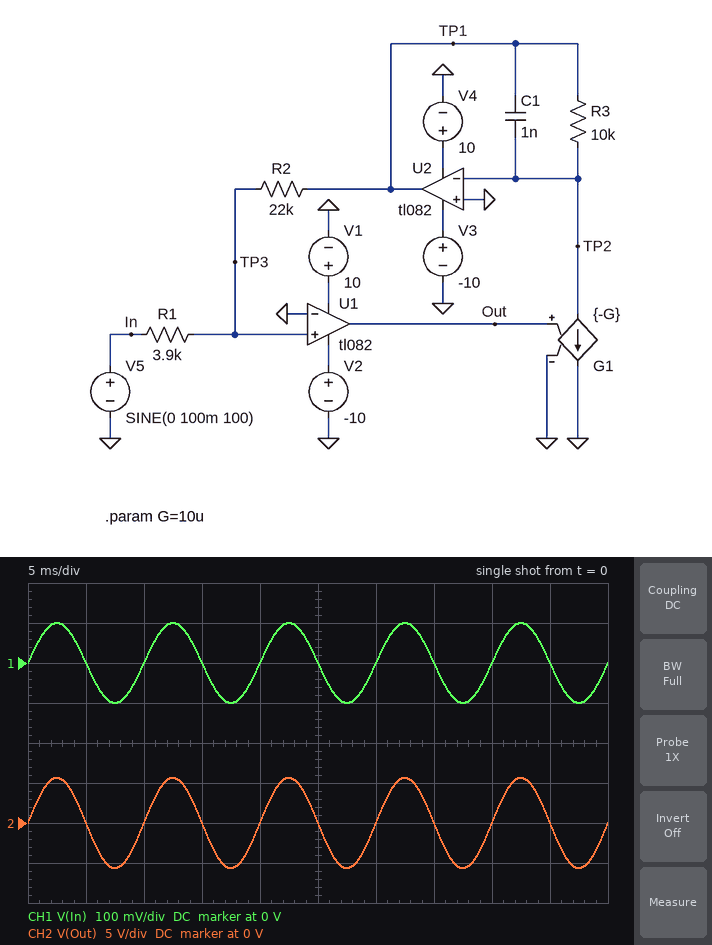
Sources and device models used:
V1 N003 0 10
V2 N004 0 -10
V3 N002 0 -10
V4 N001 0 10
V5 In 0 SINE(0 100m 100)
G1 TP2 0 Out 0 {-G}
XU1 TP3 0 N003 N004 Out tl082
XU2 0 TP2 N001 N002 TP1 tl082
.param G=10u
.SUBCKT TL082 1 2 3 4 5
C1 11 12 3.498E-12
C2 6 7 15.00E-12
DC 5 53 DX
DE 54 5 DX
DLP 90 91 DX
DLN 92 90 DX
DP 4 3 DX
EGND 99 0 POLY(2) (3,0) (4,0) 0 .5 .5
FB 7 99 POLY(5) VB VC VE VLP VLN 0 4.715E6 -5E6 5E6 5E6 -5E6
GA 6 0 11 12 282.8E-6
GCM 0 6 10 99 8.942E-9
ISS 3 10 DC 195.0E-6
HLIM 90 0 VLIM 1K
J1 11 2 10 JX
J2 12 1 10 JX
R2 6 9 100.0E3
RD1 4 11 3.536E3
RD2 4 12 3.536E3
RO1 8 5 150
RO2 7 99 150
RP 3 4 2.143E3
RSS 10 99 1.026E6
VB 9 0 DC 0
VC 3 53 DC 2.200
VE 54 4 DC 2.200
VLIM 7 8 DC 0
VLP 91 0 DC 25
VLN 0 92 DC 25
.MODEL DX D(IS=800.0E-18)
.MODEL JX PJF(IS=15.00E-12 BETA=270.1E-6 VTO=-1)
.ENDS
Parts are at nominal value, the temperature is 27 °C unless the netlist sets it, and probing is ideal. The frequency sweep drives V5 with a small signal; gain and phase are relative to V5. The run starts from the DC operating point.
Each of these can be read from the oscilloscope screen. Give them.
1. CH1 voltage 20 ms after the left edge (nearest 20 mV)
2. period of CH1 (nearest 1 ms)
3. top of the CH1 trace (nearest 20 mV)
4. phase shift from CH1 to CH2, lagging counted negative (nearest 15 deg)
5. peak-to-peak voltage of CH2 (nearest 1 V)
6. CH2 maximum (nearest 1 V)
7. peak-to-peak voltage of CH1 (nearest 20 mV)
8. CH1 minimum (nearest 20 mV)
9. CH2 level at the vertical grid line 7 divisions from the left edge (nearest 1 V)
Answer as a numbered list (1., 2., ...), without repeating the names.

1. 0 V
2. 10 ms
3. 100 mV
4. 0 deg
5. 11 V
6. 6 V
7. 200 mV
8. -100 mV
9. 0 V
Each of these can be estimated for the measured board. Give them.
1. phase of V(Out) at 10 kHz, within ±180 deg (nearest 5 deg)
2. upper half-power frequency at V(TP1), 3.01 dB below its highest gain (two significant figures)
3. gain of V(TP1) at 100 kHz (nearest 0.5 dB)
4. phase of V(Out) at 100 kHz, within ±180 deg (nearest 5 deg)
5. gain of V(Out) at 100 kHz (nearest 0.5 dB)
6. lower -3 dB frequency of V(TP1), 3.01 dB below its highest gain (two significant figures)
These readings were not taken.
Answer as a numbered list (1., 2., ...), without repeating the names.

1. 20 deg
2. 34 kHz
3. -6.0 dB
4. -90 deg
5. 30.0 dB
6. 17 kHz
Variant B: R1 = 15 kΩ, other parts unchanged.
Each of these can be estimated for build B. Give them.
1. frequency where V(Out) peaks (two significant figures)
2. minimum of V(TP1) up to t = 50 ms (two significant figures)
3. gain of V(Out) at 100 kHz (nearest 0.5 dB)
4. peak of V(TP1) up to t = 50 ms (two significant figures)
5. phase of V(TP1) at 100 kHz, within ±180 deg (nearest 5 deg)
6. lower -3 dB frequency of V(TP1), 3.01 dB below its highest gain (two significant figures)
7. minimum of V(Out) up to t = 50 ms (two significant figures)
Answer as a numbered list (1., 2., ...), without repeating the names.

1. 47 kHz
2. -150 mV
3. 28.5 dB
4. 150 mV
5. 10 deg
6. 38 kHz
7. -1.5 V
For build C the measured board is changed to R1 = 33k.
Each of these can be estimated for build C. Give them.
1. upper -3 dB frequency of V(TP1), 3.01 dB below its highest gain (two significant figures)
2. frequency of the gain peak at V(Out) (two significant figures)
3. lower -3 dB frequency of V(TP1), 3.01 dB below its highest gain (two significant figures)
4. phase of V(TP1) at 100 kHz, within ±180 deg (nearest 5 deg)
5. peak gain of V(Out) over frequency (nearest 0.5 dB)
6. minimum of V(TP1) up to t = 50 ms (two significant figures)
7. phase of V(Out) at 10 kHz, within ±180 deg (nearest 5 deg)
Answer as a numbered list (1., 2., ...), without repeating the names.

1. 63 kHz
2. 57 kHz
3. 49 kHz
4. 10 deg
5. 40.0 dB
6. -67 mV
7. 30 deg
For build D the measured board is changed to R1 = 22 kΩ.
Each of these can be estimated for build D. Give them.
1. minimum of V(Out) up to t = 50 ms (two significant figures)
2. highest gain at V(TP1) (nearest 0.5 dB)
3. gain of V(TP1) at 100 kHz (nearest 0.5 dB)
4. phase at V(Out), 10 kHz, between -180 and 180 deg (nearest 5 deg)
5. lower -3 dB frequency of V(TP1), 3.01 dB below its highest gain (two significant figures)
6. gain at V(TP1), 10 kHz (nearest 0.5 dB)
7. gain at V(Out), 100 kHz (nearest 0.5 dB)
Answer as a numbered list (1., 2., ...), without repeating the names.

1. -1.0 V
2. 11.0 dB
3. -8.5 dB
4. 30 deg
5. 43 kHz
6. 0.5 dB
7. 27.5 dB
